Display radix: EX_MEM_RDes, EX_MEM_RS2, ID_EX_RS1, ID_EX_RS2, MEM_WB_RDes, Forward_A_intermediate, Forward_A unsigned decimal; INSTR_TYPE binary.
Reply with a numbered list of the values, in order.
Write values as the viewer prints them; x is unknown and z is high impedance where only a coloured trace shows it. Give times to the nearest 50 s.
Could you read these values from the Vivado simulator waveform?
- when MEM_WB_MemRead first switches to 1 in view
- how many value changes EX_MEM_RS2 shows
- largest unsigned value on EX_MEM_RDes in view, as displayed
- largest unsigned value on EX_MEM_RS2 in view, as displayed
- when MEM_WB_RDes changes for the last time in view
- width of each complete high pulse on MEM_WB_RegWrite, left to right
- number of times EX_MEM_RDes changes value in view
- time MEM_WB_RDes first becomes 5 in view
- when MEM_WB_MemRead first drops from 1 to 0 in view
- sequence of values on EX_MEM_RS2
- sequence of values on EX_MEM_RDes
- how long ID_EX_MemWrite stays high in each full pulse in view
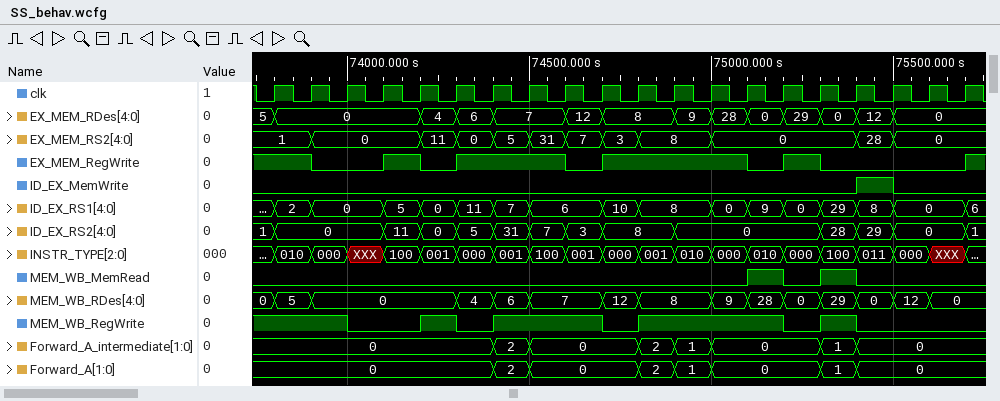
1. 75100 s
2. 11
3. 29
4. 31
5. 75600 s
6. 100 s, 300 s, 400 s, 100 s
7. 13
8. 73800 s
9. 75200 s
10. 1, 0, 11, 0, 5, 31, 7, 3, 8, 0, 28, 0
11. 5, 0, 4, 6, 7, 12, 8, 9, 28, 0, 29, 0, 12, 0
12. 100 s
